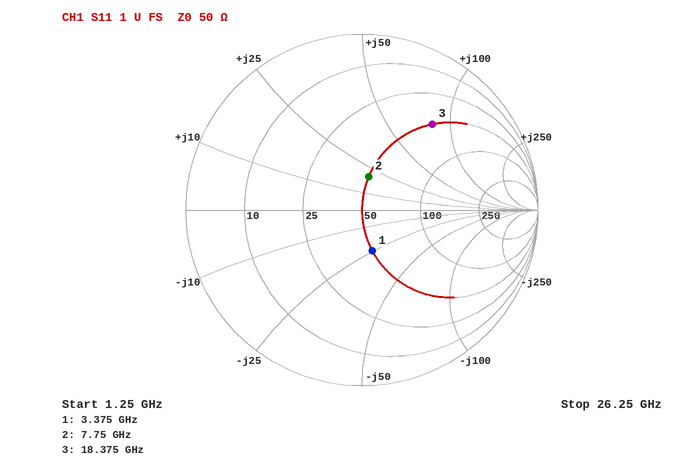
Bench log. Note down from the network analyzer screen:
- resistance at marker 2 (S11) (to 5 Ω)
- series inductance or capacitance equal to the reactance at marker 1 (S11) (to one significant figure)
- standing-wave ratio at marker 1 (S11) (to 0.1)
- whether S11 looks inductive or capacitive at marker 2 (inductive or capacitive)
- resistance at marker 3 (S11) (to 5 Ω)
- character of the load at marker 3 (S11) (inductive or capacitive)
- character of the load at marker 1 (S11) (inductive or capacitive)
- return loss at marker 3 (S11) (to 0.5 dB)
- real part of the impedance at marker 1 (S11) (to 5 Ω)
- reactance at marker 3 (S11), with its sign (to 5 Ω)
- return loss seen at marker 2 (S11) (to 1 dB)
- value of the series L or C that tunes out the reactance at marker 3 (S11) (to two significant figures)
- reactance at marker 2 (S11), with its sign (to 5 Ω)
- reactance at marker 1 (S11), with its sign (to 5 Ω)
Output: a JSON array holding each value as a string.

["50 Ω", "2 pF", "1.6", "inductive", "50 Ω", "inductive", "capacitive", "4.0 dB", "50 Ω", "+80 Ω", "14 dB", "110 fF", "+20 Ω", "-25 Ω"]
